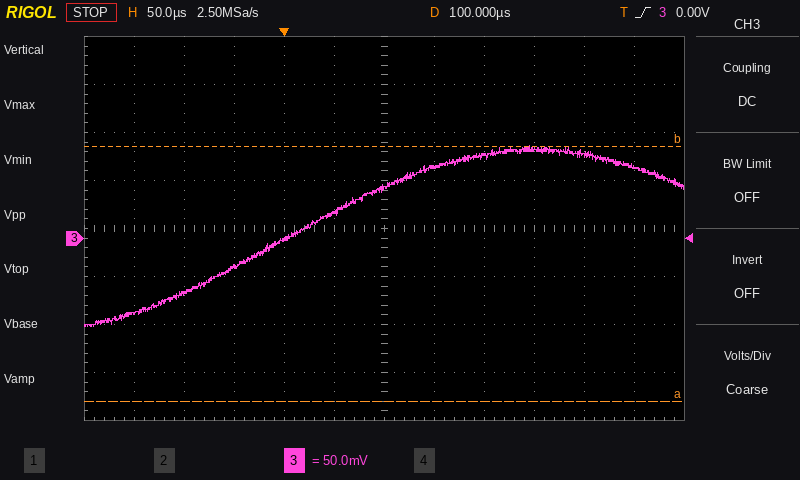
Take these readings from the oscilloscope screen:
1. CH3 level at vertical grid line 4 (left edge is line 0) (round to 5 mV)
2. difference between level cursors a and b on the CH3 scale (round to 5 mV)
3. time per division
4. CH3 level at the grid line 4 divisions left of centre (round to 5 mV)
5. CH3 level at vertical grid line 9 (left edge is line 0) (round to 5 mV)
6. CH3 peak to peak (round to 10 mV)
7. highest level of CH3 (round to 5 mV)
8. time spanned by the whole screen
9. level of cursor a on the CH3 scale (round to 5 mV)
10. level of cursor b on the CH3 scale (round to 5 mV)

0 mV
265 mV
50 µs
-55 mV
90 mV
190 mV
95 mV
600 µs
-170 mV
95 mV
